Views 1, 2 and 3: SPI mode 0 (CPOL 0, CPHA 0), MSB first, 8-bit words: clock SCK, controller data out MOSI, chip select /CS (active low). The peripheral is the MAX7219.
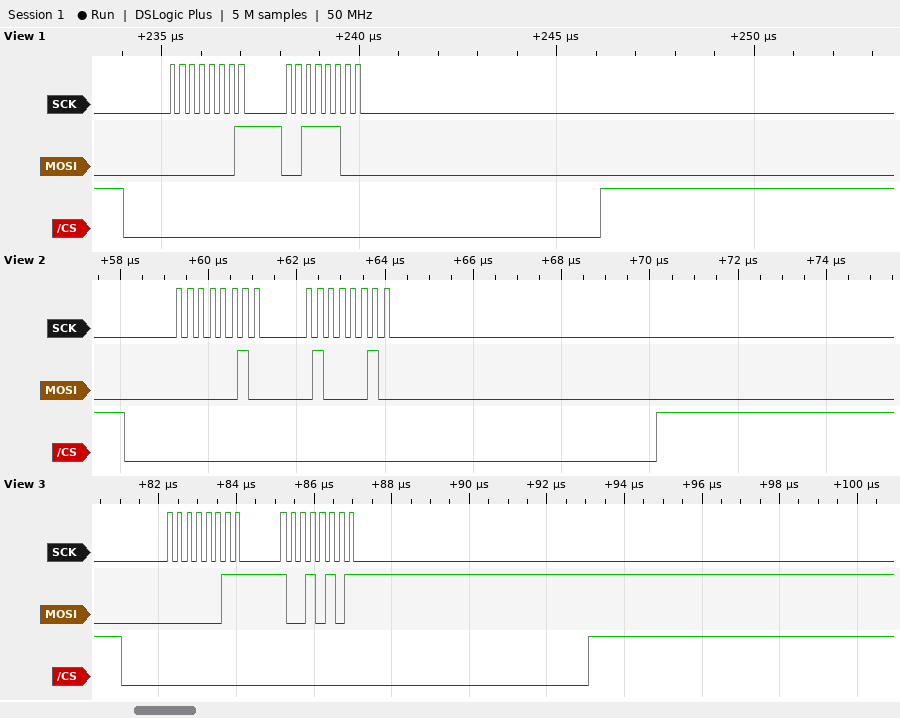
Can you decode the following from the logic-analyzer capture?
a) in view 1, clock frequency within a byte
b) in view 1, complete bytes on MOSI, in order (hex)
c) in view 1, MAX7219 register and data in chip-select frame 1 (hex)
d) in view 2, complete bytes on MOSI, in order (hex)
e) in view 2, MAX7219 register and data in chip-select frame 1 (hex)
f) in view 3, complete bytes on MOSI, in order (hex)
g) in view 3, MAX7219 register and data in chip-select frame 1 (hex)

4 MHz
01 3C
register 0x1, data 0x3C
0x02 0x42
register 0x2, data 0x42
03 95
register 0x3, data 0x95
